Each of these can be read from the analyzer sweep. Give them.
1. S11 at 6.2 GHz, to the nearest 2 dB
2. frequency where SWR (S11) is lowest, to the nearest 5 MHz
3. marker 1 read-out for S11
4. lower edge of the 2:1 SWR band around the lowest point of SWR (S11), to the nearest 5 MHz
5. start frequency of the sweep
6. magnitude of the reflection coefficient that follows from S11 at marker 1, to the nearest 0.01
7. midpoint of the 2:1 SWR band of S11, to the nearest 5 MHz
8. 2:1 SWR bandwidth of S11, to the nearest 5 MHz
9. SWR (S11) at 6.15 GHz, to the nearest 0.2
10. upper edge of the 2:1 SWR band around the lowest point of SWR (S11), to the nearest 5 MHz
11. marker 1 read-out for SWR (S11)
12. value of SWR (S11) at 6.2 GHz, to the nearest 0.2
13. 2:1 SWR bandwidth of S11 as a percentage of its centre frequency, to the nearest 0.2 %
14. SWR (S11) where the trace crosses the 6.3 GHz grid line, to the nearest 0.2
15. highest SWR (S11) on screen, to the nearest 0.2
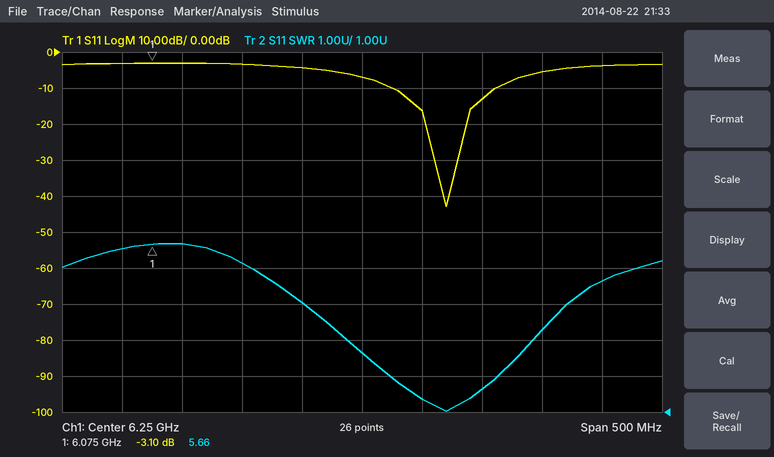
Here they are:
-4 dB
6.320 GHz
-3.10 dB
6.275 GHz
6 GHz
0.70
6.320 GHz
90 MHz
5.2
6.365 GHz
5.66
4.0
1.4 %
1.4
5.6
